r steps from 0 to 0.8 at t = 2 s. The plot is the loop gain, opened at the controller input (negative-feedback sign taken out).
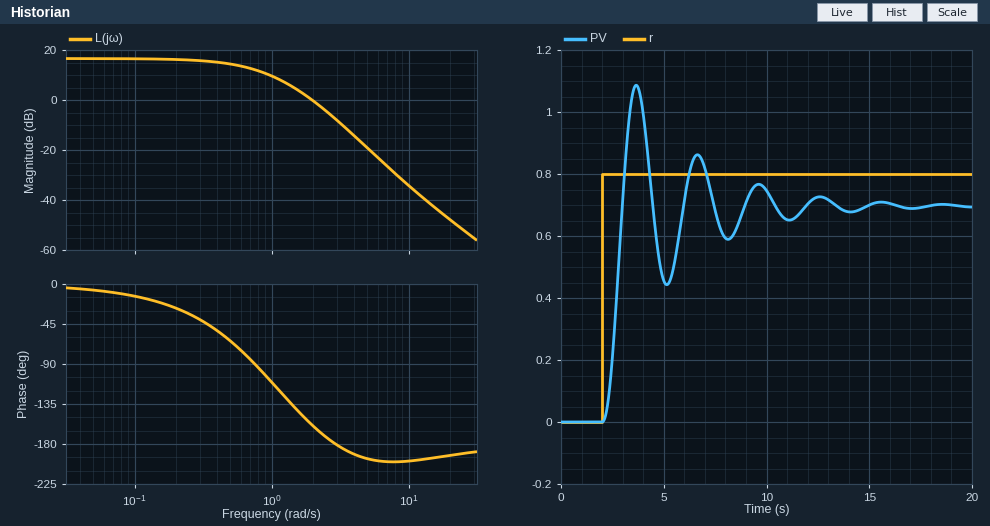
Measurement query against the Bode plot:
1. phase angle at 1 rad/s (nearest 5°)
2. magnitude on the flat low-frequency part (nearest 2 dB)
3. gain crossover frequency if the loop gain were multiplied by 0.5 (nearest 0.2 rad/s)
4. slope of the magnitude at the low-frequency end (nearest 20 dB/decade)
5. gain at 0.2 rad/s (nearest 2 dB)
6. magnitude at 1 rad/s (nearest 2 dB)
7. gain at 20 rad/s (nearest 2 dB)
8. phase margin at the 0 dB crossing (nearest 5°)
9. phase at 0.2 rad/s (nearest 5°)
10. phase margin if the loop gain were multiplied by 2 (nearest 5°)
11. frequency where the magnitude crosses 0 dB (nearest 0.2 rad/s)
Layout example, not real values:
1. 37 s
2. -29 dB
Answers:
1. -110°
2. 16 dB
3. 1.4 rad/s
4. 0 dB/decade
5. 16 dB
6. 10 dB
7. -48 dB
8. 20°
9. -25°
10. 5°
11. 2.0 rad/s
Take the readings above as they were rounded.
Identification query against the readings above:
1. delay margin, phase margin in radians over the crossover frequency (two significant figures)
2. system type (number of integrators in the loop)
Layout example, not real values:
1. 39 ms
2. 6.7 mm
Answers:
1. 0.17 s
2. 0
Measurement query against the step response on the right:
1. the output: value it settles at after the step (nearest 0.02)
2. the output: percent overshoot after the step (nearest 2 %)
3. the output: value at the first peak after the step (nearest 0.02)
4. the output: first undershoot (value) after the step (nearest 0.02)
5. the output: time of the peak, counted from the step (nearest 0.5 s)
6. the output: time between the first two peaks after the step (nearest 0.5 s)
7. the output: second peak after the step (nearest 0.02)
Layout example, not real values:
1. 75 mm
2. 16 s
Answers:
1. 0.70
2. 56 %
3. 1.08
4. 0.44
5. 1.5 s
6. 3.0 s
7. 0.86
